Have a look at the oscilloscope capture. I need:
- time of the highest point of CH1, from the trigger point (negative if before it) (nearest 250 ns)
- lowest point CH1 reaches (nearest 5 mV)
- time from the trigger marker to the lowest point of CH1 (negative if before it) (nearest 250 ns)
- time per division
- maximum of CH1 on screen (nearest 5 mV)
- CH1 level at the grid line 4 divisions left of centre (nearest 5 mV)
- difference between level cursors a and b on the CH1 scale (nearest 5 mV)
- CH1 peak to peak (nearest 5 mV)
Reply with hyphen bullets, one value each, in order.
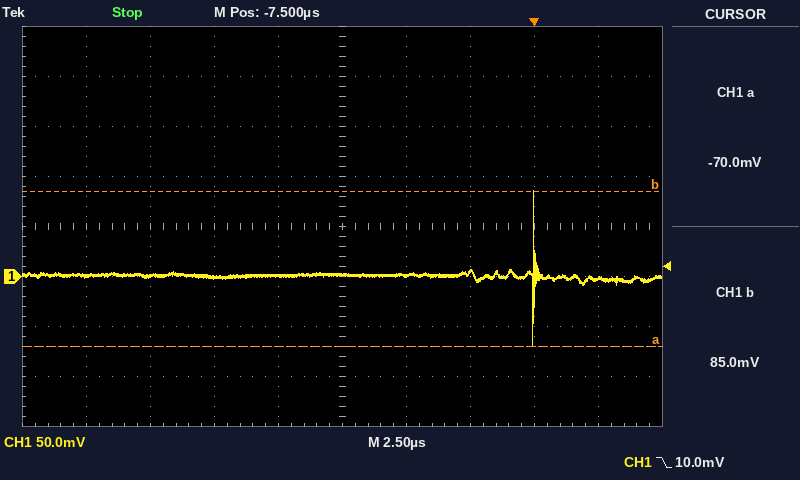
- 0.00 µs
- -70 mV
- 0.00 µs
- 2.5 µs
- 85 mV
- 0 mV
- 155 mV
- 155 mV
